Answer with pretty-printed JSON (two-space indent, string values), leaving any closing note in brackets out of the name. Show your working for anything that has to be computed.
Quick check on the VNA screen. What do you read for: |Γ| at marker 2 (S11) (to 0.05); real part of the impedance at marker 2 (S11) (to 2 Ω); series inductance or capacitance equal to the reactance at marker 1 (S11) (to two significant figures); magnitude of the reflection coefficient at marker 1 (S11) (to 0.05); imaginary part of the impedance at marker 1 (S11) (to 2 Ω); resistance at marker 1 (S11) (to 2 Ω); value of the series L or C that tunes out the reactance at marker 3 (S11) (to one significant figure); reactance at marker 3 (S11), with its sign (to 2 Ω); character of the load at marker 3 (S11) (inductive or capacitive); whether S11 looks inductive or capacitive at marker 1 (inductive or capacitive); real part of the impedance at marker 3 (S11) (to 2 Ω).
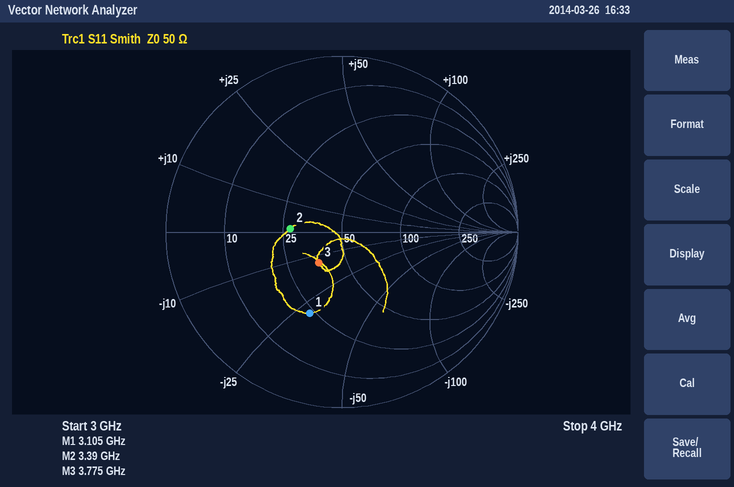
{
  "|Γ| at marker 2 (S11)": "0.30",
  "real part of the impedance at marker 2 (S11)": "28 Ω",
  "series inductance or capacitance equal to the reactance at marker 1 (S11)": "C = 1/(2π × 3.105 GHz × 28 Ω) ≈ 1.8 pF",
  "magnitude of the reflection coefficient at marker 1 (S11)": "0.50",
  "imaginary part of the impedance at marker 1 (S11)": "-28 Ω",
  "resistance at marker 1 (S11)": "24 Ω",
  "value of the series L or C that tunes out the reactance at marker 3 (S11)": "L = 14 Ω/(2π × 3.775 GHz) ≈ 590 pH, so 600 pH to one significant figure",
  "reactance at marker 3 (S11), with its sign": "-14 Ω",
  "character of the load at marker 3 (S11)": "capacitive",
  "whether S11 looks inductive or capacitive at marker 1": "capacitive",
  "real part of the impedance at marker 3 (S11)": "36 Ω"
}
